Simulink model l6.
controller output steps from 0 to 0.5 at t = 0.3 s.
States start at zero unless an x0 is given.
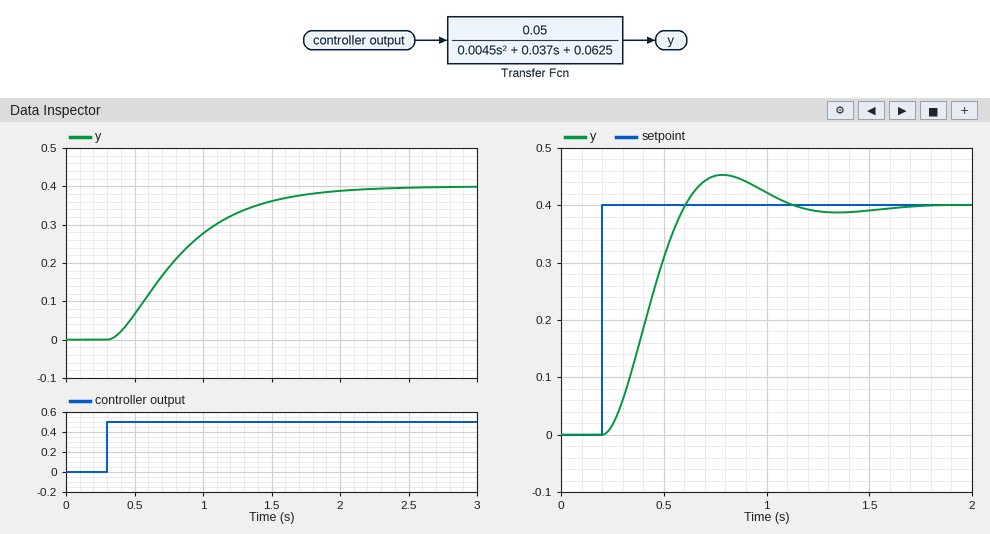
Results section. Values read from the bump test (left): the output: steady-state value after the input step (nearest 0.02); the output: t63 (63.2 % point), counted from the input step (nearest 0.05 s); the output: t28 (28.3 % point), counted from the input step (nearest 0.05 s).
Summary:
0.40
0.60 s
0.30 s
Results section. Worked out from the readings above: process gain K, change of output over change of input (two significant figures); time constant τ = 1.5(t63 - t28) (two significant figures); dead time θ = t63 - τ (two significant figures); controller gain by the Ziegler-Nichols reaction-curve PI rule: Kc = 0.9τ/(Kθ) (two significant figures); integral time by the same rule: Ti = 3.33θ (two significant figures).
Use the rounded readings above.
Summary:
0.80
0.45 s
0.15 s
3.4
0.50 s
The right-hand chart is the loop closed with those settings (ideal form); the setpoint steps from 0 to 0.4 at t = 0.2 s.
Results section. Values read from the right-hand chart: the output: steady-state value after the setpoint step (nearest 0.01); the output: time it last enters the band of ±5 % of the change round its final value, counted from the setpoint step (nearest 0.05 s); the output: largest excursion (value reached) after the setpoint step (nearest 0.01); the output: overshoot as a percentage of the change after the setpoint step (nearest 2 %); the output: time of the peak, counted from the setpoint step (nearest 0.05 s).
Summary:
0.40
0.80 s
0.45
14 %
0.60 s
